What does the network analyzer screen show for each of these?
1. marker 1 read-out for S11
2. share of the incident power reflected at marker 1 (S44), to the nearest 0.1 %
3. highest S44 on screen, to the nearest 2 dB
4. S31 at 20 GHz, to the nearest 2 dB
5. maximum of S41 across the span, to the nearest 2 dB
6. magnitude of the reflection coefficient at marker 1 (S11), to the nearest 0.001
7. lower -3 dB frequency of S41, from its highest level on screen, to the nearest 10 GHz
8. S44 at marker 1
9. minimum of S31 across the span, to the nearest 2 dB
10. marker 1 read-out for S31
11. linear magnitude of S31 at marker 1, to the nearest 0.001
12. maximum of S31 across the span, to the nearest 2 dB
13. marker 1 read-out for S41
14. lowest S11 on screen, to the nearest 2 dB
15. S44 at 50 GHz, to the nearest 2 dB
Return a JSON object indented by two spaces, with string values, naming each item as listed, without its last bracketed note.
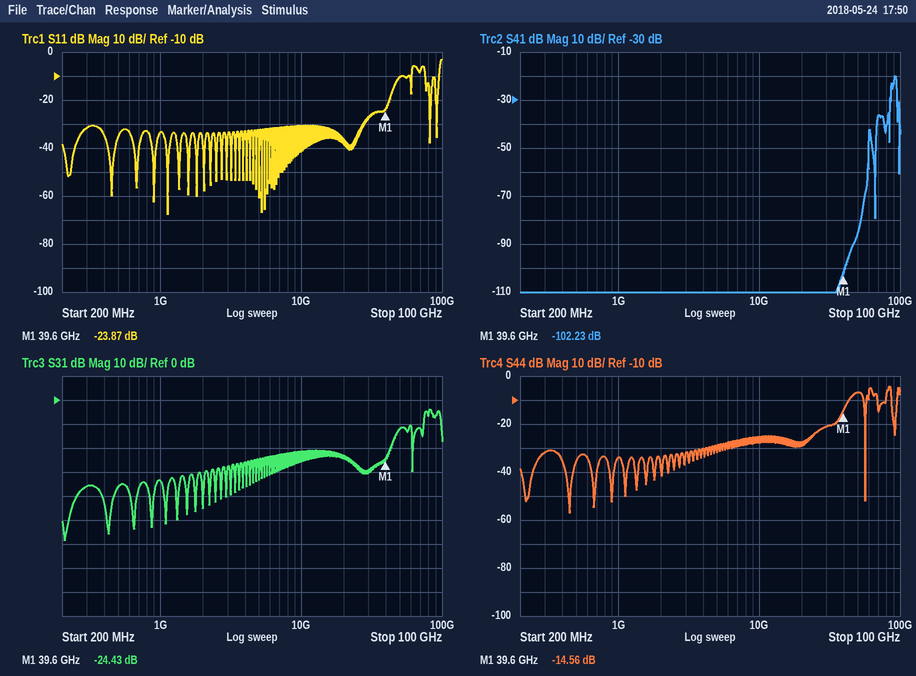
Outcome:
{
  "marker 1 read-out for S11": "-23.87 dB",
  "share of the incident power reflected at marker 1 (S44), to the nearest 0.1 %": "3.5 %",
  "highest S44 on screen, to the nearest 2 dB": "-4 dB",
  "S31 at 20 GHz, to the nearest 2 dB": "-24 dB",
  "maximum of S41 across the span, to the nearest 2 dB": "-20 dB",
  "magnitude of the reflection coefficient at marker 1 (S11), to the nearest 0.001": "0.064",
  "lower -3 dB frequency of S41, from its highest level on screen, to the nearest 10 GHz": "90 GHz",
  "S44 at marker 1": "-14.56 dB",
  "minimum of S31 across the span, to the nearest 2 dB": "-58 dB",
  "marker 1 read-out for S31": "-24.43 dB",
  "linear magnitude of S31 at marker 1, to the nearest 0.001": "0.060",
  "maximum of S31 across the span, to the nearest 2 dB": "-4 dB",
  "marker 1 read-out for S41": "-102.23 dB",
  "lowest S11 on screen, to the nearest 2 dB": "-68 dB",
  "S44 at 50 GHz, to the nearest 2 dB": "-6 dB"
}
